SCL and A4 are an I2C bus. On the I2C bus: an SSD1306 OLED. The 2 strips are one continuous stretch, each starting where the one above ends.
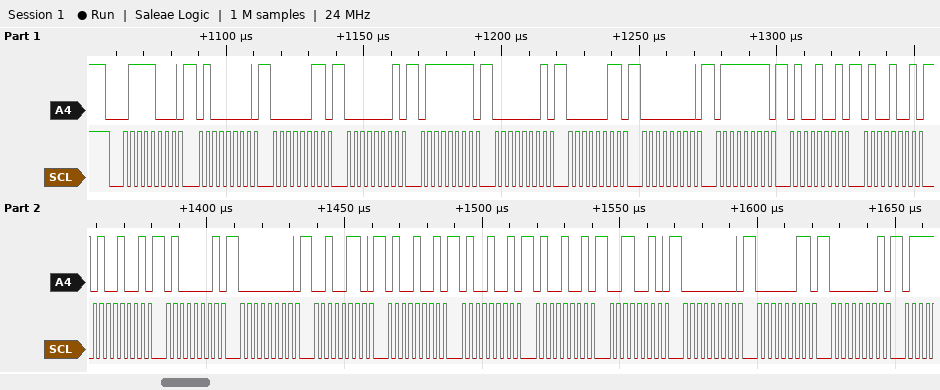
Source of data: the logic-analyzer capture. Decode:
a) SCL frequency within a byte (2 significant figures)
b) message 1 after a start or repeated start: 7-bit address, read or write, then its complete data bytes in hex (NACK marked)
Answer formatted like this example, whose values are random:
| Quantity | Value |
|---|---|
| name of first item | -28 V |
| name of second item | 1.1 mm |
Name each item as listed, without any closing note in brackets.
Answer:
| Quantity | Value |
|---|---|
| SCL frequency within a byte | 400 kHz |
| message 1 after a start or repeated start: 7-bit address, read or write, then its complete data bytes in hex | 0x3C write: 40 03 01 7F 01 03 00 7F 49 49 49 41 00 26 49 49 49 32 00 03 01 |
